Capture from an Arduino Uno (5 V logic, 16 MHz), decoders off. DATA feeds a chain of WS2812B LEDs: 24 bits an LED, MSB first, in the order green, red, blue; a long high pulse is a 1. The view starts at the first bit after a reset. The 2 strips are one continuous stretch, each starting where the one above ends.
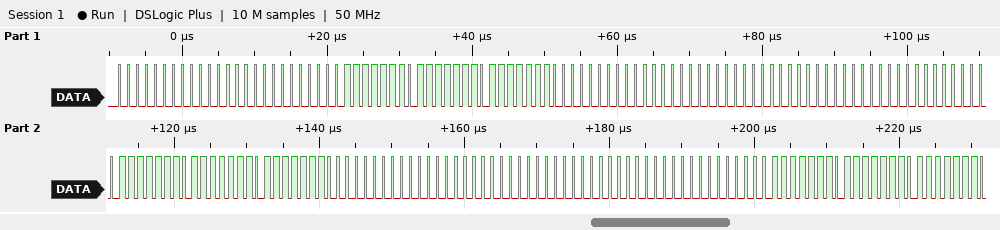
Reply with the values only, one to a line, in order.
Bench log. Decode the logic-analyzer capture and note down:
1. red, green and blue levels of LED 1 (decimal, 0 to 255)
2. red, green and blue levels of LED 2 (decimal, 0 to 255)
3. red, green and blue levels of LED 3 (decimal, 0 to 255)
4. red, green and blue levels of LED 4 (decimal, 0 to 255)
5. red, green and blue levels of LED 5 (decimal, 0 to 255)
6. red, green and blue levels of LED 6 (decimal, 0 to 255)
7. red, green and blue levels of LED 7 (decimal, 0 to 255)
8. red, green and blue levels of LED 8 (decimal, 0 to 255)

0, 0, 0
127, 127, 127
0, 0, 0
0, 0, 0
127, 127, 127
0, 0, 0
0, 0, 0
127, 127, 127
